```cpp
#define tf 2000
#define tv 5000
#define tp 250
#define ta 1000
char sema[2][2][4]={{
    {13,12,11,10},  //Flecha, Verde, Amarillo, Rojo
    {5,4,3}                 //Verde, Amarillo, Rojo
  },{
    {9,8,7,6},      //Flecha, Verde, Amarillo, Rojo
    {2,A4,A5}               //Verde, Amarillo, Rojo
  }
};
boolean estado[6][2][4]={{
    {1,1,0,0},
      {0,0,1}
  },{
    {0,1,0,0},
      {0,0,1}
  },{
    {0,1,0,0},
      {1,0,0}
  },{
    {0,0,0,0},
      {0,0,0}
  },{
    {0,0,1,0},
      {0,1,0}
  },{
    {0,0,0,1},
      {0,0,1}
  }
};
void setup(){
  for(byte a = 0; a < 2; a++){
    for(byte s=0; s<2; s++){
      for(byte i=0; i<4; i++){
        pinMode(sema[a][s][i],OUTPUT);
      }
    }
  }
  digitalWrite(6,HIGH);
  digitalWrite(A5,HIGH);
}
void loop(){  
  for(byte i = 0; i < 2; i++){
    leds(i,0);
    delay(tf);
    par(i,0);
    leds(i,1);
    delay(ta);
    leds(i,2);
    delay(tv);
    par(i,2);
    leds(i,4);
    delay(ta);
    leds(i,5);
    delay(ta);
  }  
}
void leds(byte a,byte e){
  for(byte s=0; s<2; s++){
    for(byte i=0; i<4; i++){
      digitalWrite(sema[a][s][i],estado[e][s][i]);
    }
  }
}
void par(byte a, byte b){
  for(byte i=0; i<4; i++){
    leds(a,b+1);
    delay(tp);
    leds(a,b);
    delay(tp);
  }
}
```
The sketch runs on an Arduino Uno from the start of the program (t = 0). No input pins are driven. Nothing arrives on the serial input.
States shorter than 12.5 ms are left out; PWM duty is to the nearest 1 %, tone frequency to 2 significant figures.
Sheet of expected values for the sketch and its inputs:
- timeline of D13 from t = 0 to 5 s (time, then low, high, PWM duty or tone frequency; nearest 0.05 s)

0 s high; 2 s low; 2.25 s high; 2.5 s low; 2.75 s high; 3 s low; 3.25 s high; 3.5 s low; 3.75 s high; 4 s low
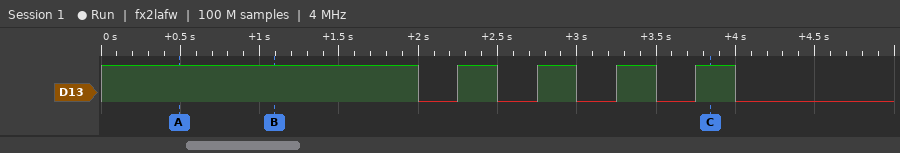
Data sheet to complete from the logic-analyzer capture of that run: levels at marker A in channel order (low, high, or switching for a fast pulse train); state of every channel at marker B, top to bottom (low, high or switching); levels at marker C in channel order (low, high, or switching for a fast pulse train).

D13 high
D13 high
D13 high
